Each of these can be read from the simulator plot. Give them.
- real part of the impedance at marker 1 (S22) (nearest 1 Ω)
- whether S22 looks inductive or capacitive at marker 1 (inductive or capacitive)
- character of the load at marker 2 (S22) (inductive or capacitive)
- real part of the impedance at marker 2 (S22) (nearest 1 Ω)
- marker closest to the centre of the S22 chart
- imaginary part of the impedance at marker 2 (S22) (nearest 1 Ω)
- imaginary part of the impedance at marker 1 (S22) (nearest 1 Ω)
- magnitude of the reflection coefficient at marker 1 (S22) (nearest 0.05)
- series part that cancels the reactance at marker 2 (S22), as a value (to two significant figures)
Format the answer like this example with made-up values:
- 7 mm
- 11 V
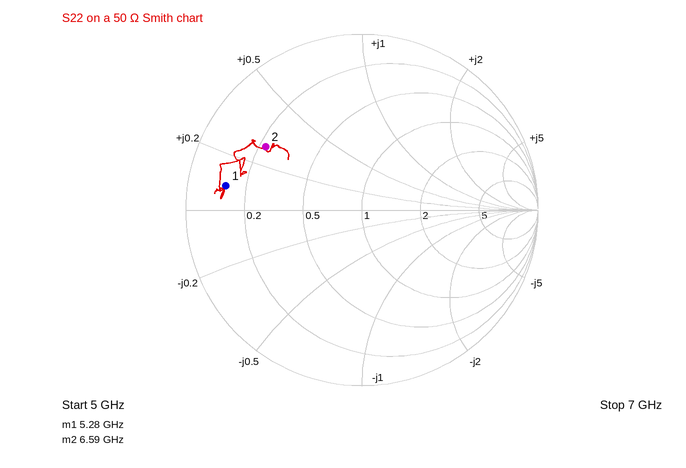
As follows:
- 6 Ω
- inductive
- inductive
- 11 Ω
- marker 2
- +14 Ω
- +4 Ω
- 0.80
- 1.7 pF
